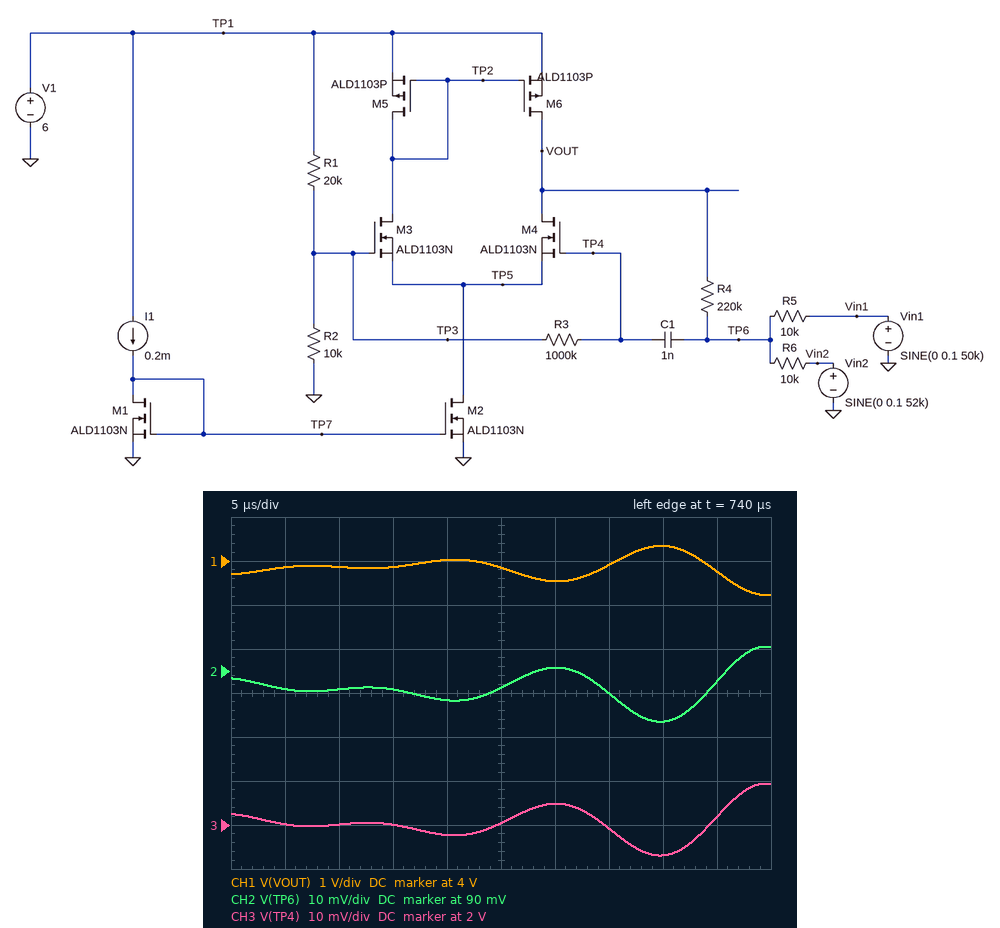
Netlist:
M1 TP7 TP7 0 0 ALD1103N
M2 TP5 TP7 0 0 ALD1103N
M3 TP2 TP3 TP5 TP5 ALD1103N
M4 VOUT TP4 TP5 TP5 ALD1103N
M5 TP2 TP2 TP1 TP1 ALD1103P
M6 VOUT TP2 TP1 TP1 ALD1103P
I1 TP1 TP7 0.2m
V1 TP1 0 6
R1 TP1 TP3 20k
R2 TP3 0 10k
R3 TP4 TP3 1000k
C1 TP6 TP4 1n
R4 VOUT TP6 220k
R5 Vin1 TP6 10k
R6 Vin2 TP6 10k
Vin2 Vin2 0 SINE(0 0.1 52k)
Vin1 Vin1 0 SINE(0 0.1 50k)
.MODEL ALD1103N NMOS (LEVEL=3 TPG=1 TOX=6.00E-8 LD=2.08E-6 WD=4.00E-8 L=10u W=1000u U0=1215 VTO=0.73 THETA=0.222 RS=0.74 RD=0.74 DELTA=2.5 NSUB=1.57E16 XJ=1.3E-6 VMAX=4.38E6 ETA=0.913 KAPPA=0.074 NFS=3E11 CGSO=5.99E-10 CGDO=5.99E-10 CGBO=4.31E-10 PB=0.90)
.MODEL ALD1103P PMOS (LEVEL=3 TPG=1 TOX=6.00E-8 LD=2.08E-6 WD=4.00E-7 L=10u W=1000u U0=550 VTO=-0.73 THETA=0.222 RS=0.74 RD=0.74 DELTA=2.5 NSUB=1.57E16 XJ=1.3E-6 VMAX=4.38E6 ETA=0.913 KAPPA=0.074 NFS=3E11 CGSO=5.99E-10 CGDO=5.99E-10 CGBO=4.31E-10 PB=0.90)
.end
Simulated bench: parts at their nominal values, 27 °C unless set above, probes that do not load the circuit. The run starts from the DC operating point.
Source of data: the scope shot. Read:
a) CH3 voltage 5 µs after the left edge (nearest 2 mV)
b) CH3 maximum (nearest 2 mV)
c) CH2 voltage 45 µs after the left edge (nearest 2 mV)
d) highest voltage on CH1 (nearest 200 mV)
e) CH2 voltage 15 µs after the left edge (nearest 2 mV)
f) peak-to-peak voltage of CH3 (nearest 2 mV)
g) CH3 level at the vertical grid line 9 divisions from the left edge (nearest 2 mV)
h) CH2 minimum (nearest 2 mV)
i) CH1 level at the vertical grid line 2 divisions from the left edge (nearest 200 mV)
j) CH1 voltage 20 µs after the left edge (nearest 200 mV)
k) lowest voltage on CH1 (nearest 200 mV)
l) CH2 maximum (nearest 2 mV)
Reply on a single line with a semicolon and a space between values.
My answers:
2.000 V; 2.010 V; 88 mV; 4.4 V; 86 mV; 16 mV; 2.002 V; 78 mV; 3.8 V; 4.0 V; 3.2 V; 96 mV
